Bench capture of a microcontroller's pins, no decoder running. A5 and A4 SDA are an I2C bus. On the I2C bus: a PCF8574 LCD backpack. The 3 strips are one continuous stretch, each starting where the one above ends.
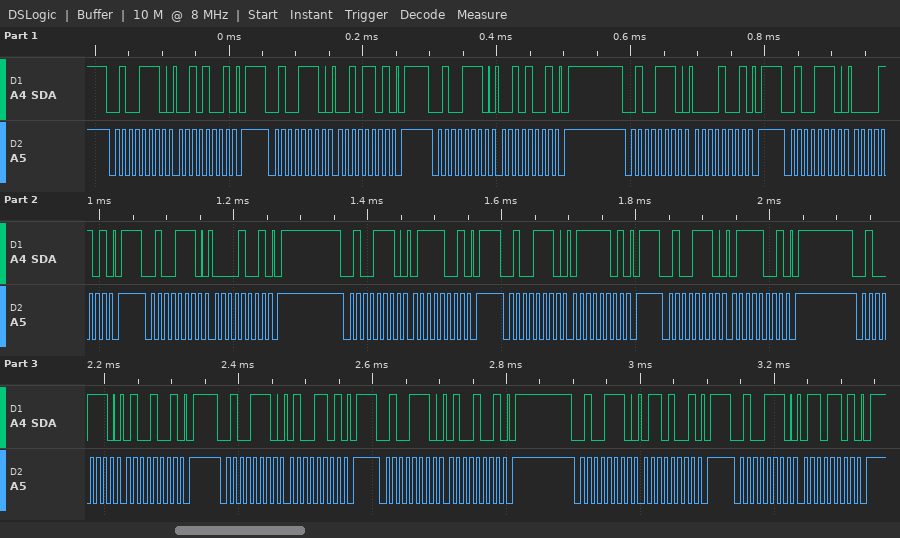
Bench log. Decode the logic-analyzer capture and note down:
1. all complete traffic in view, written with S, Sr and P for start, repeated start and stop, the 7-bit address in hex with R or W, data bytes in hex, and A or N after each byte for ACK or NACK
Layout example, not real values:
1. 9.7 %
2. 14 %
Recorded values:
1. S 27W A 29 A P S 27W A 2D A P S 27W A 29 A P S 27W A 09 A P S 27W A 0D A P S 27W A 09 A P S 27W A 79 A P S 27W A 7D A P S 27W A 79 A P S 27W A 49 A P S 27W A 4D A P S 27W A 49 A P S 27W A 69 A P S 27W A 6D A P
